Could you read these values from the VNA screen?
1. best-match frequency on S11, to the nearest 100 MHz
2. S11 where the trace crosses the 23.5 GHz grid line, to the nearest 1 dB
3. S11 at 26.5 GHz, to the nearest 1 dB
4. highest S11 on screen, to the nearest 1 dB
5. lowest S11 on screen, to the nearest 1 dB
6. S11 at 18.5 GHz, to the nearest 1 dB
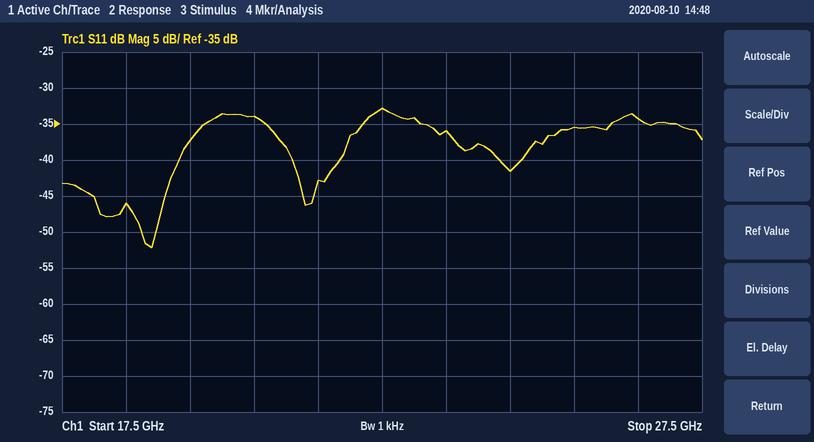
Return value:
18.9 GHz
-36 dB
-34 dB
-33 dB
-52 dB
-46 dB
